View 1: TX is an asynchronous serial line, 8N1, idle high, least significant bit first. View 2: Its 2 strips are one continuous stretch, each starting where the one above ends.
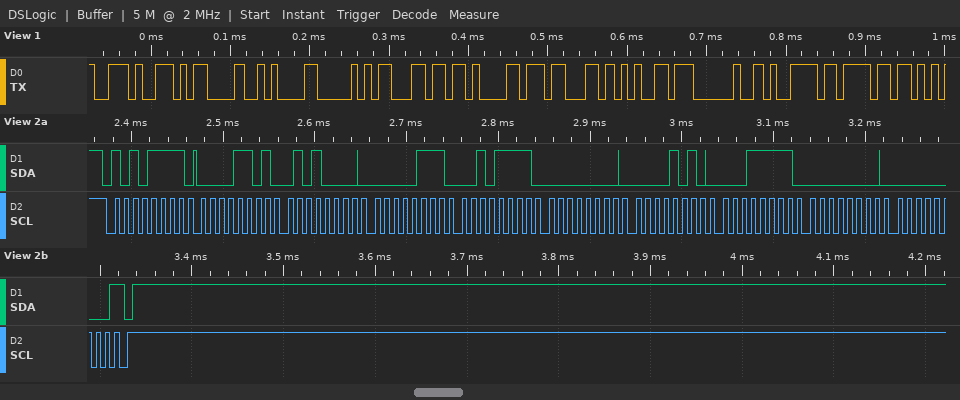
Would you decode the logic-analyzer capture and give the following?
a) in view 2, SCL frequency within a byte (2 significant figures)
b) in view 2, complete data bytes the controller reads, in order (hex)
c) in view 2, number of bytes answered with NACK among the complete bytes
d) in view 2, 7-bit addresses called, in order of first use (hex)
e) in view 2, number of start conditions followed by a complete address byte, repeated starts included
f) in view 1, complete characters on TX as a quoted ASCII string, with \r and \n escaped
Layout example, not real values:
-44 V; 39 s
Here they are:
100 kHz; 0D 50 07 2F 00 0A 1F 00 00; 1; 0x57; 1; ".\r\nPlace yo"
